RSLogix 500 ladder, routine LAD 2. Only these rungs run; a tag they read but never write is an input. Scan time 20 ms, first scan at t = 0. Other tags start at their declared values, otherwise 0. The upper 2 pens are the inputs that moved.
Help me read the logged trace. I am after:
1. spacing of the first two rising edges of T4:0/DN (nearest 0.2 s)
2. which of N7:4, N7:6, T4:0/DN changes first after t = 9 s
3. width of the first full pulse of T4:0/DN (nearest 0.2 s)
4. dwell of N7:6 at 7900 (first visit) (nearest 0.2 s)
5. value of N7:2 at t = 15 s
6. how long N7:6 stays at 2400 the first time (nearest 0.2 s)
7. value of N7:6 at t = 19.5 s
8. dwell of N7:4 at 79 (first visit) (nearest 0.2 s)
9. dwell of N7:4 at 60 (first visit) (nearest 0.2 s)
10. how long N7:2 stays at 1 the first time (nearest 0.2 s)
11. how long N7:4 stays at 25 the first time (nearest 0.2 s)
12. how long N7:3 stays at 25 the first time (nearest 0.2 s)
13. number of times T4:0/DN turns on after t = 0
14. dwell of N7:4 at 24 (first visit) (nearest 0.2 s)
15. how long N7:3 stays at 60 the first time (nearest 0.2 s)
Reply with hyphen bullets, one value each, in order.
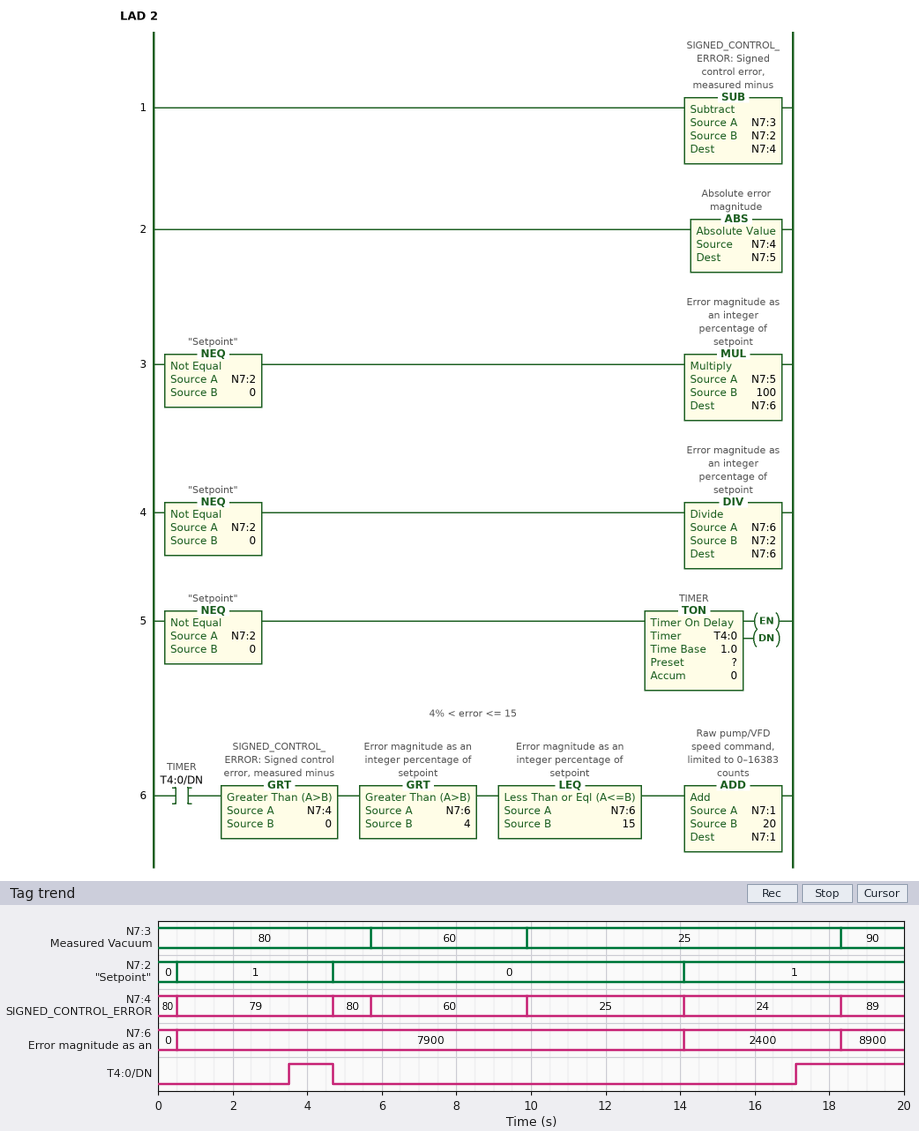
- 13.6 s
- N7:4
- 1.2 s
- 13.6 s
- 1
- 4.2 s
- 8900
- 4.2 s
- 4.2 s
- 4.2 s
- 4.2 s
- 8.4 s
- 2
- 4.2 s
- 4.2 s
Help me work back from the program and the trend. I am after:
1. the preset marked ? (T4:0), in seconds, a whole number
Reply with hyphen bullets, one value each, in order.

- 3 s
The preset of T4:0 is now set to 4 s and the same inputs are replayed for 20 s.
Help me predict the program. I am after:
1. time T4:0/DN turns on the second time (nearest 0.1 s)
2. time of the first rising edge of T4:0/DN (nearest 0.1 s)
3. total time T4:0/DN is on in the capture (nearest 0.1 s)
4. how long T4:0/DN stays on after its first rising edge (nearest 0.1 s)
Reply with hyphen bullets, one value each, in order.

- 18.1 s
- 4.5 s
- 2.1 s
- 0.2 s
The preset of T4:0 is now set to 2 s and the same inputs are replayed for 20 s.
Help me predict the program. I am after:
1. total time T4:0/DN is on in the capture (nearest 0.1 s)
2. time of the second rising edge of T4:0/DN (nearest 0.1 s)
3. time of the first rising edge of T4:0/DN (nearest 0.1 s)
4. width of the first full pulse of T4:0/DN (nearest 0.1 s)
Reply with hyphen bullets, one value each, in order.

- 6.1 s
- 16.1 s
- 2.5 s
- 2.2 s
